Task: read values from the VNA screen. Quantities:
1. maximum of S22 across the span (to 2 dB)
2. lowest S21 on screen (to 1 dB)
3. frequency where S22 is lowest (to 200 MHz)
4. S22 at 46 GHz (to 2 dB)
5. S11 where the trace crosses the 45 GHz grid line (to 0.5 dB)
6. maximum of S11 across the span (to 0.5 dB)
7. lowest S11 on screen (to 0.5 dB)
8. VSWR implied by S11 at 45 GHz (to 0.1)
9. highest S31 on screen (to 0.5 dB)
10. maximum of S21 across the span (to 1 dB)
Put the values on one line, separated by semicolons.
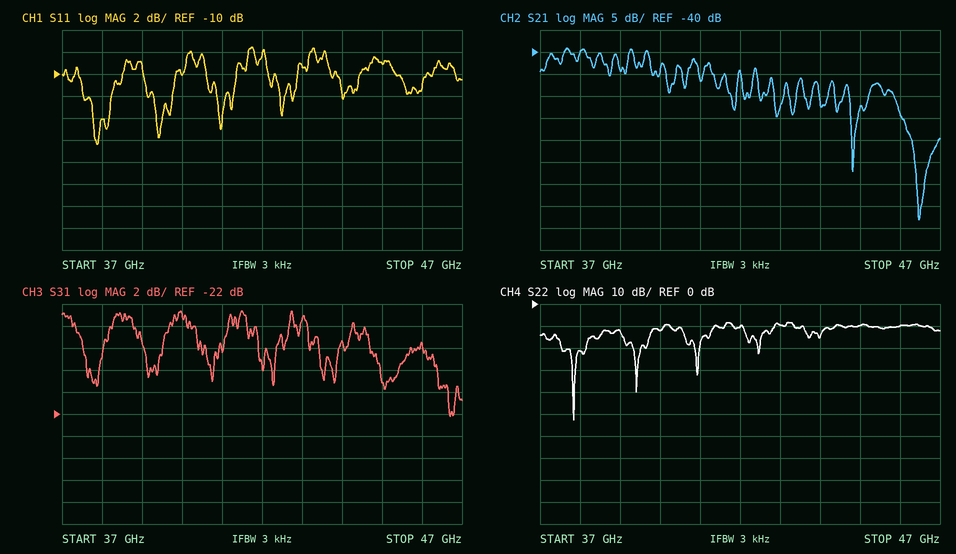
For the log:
-8 dB; -78 dB; 37.8 GHz; -10 dB; -9.0 dB; -7.5 dB; -16.5 dB; 2.1; -12.5 dB; -39 dB
